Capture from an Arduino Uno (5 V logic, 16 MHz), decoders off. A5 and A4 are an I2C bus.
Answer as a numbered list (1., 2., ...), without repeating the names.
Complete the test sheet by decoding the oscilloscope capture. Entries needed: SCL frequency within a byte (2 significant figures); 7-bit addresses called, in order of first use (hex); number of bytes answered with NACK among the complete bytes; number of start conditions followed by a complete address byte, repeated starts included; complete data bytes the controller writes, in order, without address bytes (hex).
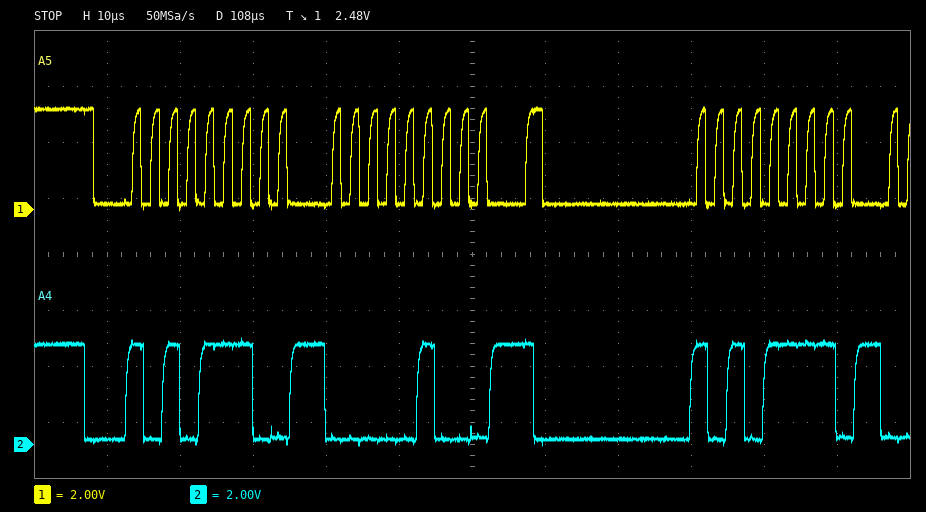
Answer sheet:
1. 400 kHz
2. 0x57
3. 0
4. 2
5. 04
